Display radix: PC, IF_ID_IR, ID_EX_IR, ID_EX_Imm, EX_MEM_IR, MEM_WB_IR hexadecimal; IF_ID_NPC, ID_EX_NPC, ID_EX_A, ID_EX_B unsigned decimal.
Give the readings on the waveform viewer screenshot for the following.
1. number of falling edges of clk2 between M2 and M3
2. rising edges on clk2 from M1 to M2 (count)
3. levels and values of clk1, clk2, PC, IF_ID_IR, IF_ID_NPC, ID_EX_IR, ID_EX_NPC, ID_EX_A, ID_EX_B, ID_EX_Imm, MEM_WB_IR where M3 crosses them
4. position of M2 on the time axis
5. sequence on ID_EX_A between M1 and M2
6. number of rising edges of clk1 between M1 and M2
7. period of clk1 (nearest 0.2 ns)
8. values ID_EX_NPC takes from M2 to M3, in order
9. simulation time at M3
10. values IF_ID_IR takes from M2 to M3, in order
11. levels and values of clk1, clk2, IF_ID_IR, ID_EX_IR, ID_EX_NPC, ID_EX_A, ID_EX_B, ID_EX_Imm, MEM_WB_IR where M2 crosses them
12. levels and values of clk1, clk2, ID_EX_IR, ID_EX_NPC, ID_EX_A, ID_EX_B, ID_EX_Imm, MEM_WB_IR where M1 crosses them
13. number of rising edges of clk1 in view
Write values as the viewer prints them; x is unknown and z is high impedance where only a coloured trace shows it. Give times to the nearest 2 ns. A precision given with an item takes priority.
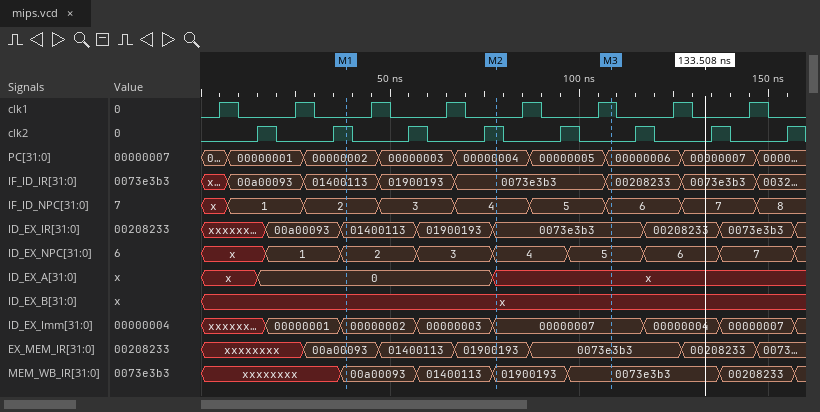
2
2
clk1=1, clk2=0, PC=00000006, IF_ID_IR=00208233, IF_ID_NPC=6, ID_EX_IR=0073e3b3, ID_EX_NPC=5, ID_EX_A=x, ID_EX_B=x, ID_EX_Imm=00000007, MEM_WB_IR=0073e3b3
78 ns
0, x
2
20 ns
4, 5
108 ns
0073e3b3, 00208233
clk1=0, clk2=1, IF_ID_IR=0073e3b3, ID_EX_IR=0073e3b3, ID_EX_NPC=4, ID_EX_A=x, ID_EX_B=x, ID_EX_Imm=00000007, MEM_WB_IR=01900193
clk1=0, clk2=1, ID_EX_IR=01400113, ID_EX_NPC=2, ID_EX_A=0, ID_EX_B=x, ID_EX_Imm=00000002, MEM_WB_IR=00a00093
8
